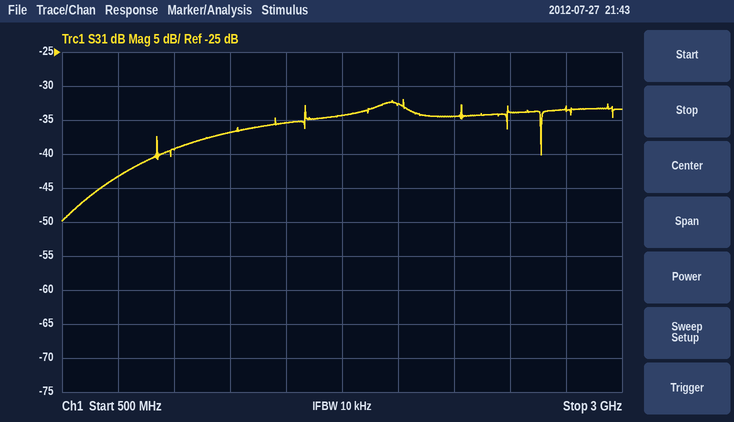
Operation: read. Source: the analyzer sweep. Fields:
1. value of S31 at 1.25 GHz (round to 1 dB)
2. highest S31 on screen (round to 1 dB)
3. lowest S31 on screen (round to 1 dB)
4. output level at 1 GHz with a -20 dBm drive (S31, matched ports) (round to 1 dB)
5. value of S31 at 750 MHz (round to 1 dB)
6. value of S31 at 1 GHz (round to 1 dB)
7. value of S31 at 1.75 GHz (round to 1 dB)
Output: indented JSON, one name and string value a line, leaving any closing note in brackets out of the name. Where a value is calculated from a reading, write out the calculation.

{
  "value of S31 at 1.25 GHz": "-37 dB",
  "highest S31 on screen": "-32 dB",
  "lowest S31 on screen": "-50 dB",
  "output level at 1 GHz with a -20 dBm drive (S31, matched ports)": "-20 dBm + (-39 dB) = -59 dBm",
  "value of S31 at 750 MHz": "-43 dB",
  "value of S31 at 1 GHz": "-39 dB",
  "value of S31 at 1.75 GHz": "-34 dB"
}
